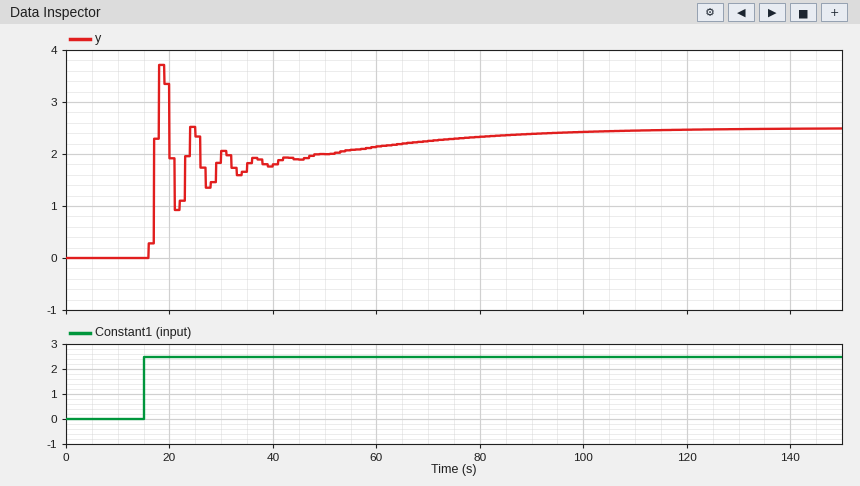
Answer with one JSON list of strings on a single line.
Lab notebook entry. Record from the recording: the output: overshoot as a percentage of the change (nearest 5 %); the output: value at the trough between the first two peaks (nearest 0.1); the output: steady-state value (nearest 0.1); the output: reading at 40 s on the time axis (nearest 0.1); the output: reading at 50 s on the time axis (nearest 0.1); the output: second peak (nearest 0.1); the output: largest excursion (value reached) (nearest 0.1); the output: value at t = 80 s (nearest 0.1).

["50 %", "0.9", "2.5", "1.8", "2.0", "2.5", "3.7", "2.3"]
